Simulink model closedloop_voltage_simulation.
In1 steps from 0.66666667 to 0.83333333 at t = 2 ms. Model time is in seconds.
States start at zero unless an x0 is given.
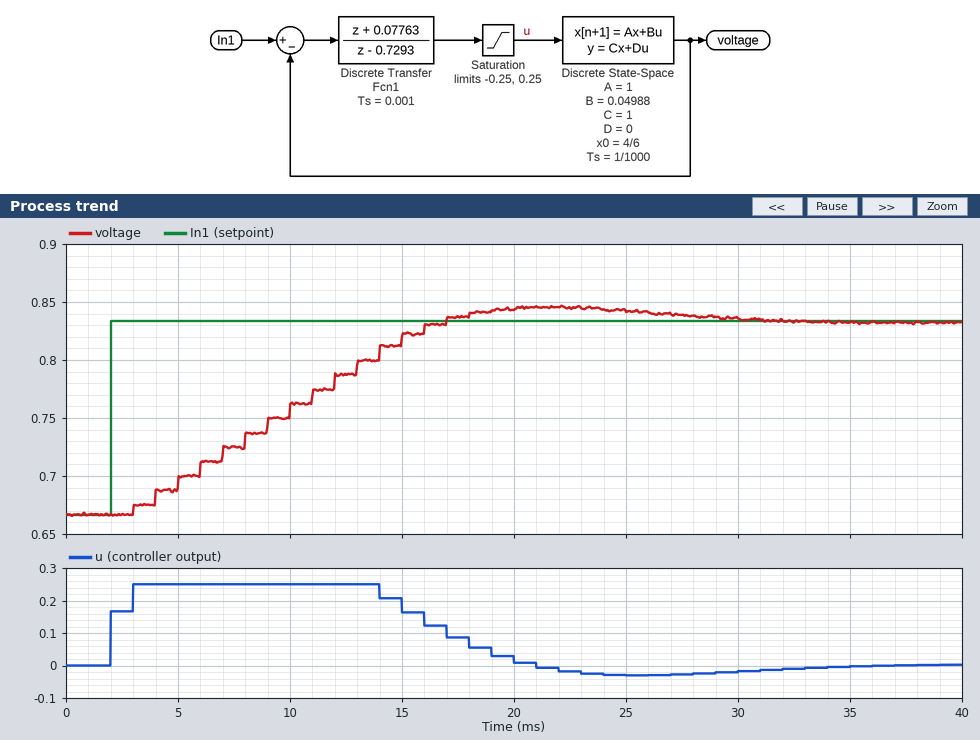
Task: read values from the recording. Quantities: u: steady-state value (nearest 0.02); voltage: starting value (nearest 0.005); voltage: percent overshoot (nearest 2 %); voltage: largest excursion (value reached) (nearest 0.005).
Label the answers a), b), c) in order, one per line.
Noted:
a) 0.00
b) 0.665
c) 8 %
d) 0.845
